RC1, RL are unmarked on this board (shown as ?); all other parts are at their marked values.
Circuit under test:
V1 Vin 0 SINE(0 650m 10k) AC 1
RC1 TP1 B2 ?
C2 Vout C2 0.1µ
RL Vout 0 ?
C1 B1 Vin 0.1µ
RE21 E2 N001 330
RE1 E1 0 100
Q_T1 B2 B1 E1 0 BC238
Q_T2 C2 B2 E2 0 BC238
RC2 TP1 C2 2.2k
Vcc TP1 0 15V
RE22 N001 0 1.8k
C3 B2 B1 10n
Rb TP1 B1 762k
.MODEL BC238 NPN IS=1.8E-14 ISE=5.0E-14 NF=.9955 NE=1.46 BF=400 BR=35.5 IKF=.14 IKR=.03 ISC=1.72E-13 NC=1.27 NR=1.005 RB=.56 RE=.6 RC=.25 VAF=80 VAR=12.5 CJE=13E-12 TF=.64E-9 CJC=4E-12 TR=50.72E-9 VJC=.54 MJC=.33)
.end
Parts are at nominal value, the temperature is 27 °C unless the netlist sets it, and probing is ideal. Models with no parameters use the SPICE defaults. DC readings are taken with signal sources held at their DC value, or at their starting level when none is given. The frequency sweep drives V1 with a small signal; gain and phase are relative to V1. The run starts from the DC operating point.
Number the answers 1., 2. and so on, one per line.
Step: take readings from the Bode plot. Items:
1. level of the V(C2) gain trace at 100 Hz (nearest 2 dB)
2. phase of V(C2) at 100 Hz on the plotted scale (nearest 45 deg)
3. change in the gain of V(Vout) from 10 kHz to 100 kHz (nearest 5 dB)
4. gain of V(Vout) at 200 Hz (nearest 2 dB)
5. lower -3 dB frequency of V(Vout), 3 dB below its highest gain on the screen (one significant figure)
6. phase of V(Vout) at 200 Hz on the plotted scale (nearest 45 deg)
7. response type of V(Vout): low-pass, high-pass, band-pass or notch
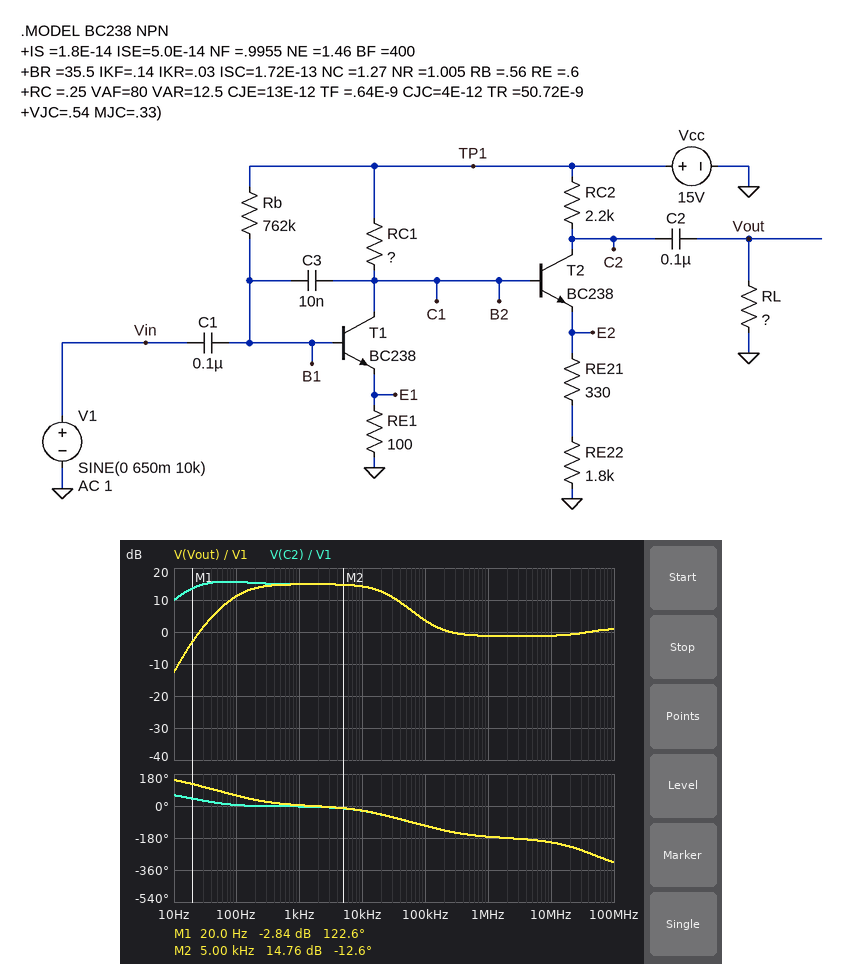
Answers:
1. 16 dB
2. 0 deg
3. -10 dB
4. 14 dB
5. 100 Hz
6. 45 deg
7. band-pass
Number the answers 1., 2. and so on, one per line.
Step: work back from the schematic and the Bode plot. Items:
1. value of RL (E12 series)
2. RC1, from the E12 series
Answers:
1. 12 kΩ
2. 2.2 kΩ
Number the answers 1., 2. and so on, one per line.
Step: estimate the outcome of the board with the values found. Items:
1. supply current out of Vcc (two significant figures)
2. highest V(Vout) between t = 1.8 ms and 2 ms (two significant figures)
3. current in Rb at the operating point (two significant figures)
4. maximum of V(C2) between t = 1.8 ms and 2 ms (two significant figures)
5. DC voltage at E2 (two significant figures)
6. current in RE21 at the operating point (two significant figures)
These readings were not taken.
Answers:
1. 6.6 mA
2. 2.9 V
3. 18 µA
4. 14 V
5. 2.4 V
6. 1.1 mA
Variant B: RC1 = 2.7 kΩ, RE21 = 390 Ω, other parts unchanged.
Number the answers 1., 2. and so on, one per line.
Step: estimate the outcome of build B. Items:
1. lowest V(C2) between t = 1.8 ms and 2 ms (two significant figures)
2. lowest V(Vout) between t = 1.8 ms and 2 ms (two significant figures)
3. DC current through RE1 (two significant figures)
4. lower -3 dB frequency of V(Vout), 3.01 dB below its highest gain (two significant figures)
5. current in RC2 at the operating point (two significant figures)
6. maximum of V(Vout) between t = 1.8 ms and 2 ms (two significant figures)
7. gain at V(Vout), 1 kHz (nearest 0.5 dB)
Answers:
1. 7.9 V
2. -4.1 V
3. 5.3 mA
4. 120 Hz
5. 110 µA
6. 2.5 V
7. 14.5 dB
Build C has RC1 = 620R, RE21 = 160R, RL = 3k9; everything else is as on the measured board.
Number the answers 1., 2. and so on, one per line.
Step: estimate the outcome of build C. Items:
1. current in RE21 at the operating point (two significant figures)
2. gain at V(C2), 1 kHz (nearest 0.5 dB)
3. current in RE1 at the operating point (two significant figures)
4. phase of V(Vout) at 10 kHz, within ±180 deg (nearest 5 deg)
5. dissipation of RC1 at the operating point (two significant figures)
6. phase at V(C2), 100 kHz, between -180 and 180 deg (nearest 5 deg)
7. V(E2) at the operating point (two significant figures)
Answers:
1. 4.7 mA
2. 7.5 dB
3. 5.9 mA
4. 170 deg
5. 40 mW
6. 90 deg
7. 9.3 V
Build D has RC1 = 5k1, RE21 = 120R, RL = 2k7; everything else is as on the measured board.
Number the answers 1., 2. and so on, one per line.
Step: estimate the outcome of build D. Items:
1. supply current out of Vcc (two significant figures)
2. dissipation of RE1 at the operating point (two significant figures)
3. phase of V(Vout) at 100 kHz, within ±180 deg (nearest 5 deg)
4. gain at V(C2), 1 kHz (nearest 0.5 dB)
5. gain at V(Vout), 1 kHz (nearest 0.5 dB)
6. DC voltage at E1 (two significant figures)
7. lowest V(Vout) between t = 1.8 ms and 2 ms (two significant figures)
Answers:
1. 2.9 mA
2. 830 µW
3. -130 deg
4. -43.0 dB
5. -44.5 dB
6. 290 mV
7. -2.7 V
